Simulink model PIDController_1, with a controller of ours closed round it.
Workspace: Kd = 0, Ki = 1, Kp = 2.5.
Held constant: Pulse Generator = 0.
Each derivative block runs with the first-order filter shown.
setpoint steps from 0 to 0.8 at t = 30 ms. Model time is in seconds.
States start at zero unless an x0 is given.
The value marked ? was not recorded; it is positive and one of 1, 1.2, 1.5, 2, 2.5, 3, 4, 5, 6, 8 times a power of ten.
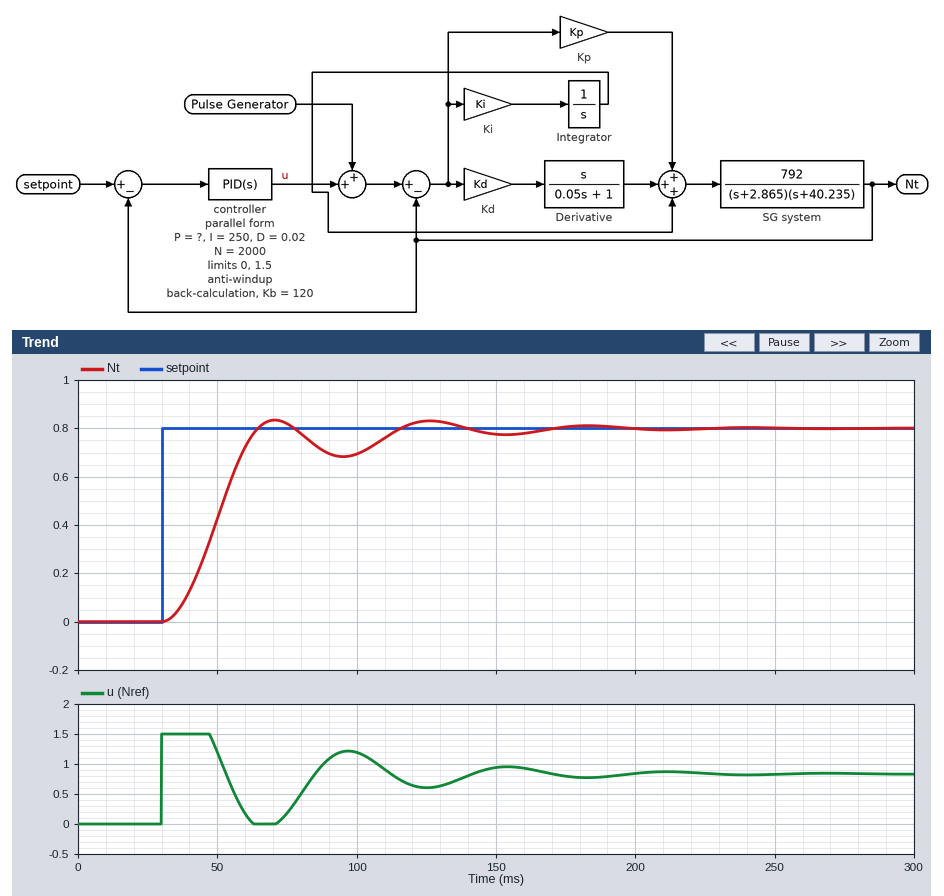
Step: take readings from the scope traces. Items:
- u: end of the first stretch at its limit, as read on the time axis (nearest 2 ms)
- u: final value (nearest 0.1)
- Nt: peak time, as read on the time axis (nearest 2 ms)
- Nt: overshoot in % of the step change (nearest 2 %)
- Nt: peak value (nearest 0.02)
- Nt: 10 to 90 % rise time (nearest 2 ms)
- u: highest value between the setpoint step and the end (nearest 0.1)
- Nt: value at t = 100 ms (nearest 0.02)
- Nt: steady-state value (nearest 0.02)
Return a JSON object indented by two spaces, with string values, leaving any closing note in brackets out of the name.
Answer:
{
  "u: end of the first stretch at its limit, as read on the time axis": "48 ms",
  "u: final value": "0.8",
  "Nt: peak time, as read on the time axis": "70 ms",
  "Nt: overshoot in % of the step change": "4 %",
  "Nt: peak value": "0.84",
  "Nt: 10 to 90 % rise time": "22 ms",
  "u: highest value between the setpoint step and the end": "1.5",
  "Nt: value at t = 100 ms": "0.70",
  "Nt: steady-state value": "0.80"
}
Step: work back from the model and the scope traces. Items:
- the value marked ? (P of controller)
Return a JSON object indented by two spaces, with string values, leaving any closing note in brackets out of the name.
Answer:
{
  "the value marked ?": "6"
}
